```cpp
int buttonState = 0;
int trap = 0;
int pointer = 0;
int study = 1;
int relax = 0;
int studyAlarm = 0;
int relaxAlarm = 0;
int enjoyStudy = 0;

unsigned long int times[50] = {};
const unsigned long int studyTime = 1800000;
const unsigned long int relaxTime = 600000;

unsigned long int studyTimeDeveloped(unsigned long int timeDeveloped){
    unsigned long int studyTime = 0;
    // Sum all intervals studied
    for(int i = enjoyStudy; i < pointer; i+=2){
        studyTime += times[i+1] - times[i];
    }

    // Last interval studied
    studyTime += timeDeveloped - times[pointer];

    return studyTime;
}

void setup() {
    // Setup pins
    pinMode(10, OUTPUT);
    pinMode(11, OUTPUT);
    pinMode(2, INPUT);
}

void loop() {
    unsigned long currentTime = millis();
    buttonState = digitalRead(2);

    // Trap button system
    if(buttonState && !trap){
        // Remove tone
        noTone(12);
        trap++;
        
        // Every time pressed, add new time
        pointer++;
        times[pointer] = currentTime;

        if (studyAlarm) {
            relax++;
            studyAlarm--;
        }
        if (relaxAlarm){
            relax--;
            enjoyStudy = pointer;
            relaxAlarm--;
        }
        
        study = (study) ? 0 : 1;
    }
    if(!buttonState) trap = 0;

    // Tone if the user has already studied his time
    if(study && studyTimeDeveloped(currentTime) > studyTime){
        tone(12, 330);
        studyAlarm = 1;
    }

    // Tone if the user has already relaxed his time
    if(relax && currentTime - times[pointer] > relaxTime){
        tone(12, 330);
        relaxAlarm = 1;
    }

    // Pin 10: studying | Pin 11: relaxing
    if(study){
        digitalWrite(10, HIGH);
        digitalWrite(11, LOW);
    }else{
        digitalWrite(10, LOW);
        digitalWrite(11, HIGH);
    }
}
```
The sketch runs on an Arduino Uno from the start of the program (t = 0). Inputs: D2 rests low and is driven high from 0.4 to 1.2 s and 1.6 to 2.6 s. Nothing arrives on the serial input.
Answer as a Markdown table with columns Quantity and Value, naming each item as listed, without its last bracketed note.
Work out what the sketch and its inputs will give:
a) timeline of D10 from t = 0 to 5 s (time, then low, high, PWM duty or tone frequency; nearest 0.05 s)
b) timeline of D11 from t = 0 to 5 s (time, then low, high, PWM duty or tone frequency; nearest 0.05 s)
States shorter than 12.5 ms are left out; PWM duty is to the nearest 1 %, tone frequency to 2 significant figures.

| Quantity | Value |
|---|---|
| timeline of D10 from t = 0 to 5 s | 0 s high; 0.4 s low; 1.6 s high |
| timeline of D11 from t = 0 to 5 s | 0 s low; 0.4 s high; 1.6 s low |
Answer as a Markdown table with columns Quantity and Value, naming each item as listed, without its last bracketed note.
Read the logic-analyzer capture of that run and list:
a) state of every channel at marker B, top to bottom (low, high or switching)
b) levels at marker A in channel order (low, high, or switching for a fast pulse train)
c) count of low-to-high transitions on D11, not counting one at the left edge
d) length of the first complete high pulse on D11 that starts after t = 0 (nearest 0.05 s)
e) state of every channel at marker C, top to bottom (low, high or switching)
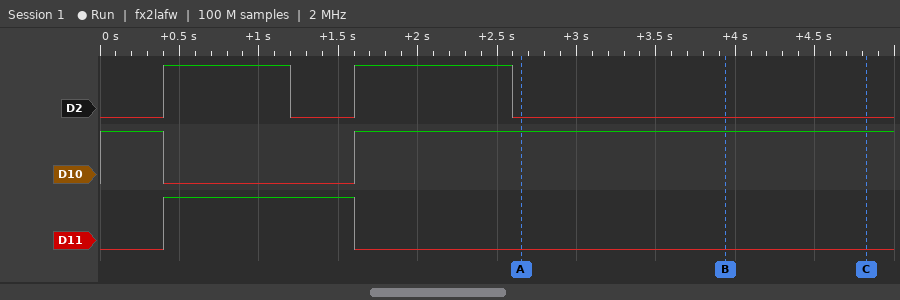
| Quantity | Value |
|---|---|
| state of every channel at marker B, top to bottom | D2 low, D10 high, D11 low |
| levels at marker A in channel order | D2 low, D10 high, D11 low |
| count of low-to-high transitions on D11, not counting one at the left edge | 1 |
| length of the first complete high pulse on D11 that starts after t = 0 | 1.20 s |
| state of every channel at marker C, top to bottom | D2 low, D10 high, D11 low |
